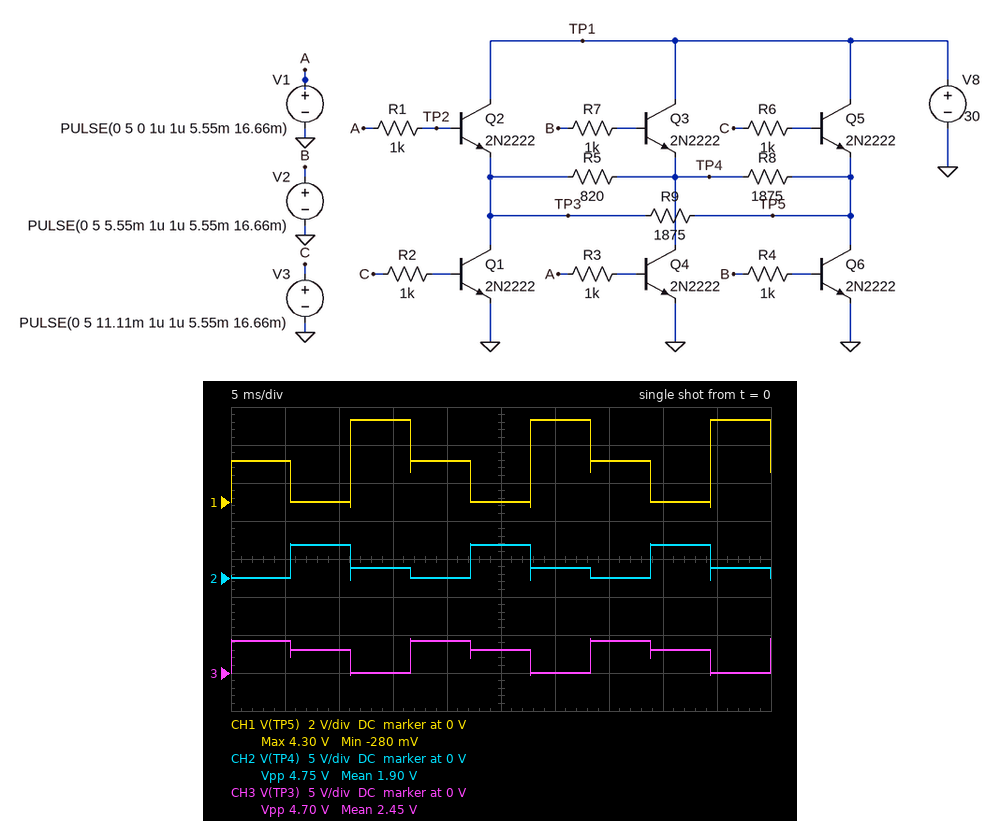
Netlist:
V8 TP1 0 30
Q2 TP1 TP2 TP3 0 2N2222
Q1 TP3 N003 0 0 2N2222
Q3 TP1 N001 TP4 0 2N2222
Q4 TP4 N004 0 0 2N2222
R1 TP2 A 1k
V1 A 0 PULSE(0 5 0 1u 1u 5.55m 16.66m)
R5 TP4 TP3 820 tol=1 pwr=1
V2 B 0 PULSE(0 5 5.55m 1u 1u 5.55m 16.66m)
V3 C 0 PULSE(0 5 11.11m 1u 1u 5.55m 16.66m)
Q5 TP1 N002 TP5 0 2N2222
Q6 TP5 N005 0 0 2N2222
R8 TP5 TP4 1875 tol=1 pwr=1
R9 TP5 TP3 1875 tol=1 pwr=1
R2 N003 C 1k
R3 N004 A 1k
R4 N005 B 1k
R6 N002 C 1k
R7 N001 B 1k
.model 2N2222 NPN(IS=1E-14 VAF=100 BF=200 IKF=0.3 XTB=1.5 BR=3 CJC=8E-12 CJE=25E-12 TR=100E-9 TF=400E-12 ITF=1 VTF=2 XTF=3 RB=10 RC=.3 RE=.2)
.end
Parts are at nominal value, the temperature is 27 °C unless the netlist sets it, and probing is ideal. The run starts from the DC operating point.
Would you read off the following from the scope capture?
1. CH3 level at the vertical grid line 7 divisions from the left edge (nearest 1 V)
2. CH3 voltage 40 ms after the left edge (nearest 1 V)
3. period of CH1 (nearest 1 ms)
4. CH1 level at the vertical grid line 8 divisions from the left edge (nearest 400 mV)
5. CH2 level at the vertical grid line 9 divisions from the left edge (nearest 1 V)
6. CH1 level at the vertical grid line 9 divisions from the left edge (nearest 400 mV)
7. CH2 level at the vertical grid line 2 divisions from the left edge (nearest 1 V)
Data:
4 V
3 V
17 ms
0 V
1 V
4.4 V
4 V
